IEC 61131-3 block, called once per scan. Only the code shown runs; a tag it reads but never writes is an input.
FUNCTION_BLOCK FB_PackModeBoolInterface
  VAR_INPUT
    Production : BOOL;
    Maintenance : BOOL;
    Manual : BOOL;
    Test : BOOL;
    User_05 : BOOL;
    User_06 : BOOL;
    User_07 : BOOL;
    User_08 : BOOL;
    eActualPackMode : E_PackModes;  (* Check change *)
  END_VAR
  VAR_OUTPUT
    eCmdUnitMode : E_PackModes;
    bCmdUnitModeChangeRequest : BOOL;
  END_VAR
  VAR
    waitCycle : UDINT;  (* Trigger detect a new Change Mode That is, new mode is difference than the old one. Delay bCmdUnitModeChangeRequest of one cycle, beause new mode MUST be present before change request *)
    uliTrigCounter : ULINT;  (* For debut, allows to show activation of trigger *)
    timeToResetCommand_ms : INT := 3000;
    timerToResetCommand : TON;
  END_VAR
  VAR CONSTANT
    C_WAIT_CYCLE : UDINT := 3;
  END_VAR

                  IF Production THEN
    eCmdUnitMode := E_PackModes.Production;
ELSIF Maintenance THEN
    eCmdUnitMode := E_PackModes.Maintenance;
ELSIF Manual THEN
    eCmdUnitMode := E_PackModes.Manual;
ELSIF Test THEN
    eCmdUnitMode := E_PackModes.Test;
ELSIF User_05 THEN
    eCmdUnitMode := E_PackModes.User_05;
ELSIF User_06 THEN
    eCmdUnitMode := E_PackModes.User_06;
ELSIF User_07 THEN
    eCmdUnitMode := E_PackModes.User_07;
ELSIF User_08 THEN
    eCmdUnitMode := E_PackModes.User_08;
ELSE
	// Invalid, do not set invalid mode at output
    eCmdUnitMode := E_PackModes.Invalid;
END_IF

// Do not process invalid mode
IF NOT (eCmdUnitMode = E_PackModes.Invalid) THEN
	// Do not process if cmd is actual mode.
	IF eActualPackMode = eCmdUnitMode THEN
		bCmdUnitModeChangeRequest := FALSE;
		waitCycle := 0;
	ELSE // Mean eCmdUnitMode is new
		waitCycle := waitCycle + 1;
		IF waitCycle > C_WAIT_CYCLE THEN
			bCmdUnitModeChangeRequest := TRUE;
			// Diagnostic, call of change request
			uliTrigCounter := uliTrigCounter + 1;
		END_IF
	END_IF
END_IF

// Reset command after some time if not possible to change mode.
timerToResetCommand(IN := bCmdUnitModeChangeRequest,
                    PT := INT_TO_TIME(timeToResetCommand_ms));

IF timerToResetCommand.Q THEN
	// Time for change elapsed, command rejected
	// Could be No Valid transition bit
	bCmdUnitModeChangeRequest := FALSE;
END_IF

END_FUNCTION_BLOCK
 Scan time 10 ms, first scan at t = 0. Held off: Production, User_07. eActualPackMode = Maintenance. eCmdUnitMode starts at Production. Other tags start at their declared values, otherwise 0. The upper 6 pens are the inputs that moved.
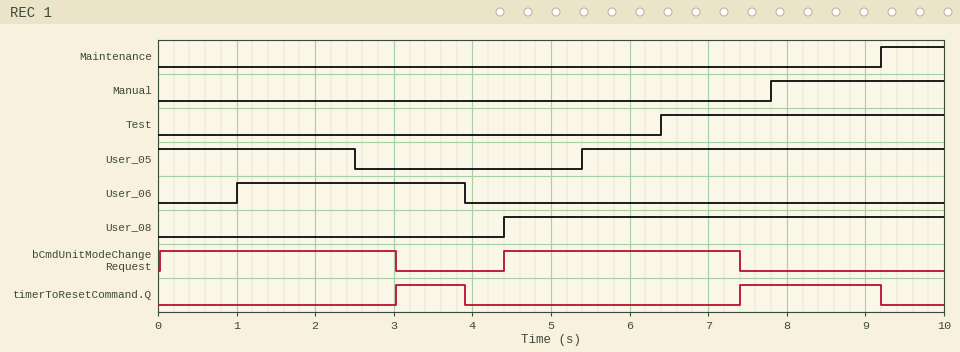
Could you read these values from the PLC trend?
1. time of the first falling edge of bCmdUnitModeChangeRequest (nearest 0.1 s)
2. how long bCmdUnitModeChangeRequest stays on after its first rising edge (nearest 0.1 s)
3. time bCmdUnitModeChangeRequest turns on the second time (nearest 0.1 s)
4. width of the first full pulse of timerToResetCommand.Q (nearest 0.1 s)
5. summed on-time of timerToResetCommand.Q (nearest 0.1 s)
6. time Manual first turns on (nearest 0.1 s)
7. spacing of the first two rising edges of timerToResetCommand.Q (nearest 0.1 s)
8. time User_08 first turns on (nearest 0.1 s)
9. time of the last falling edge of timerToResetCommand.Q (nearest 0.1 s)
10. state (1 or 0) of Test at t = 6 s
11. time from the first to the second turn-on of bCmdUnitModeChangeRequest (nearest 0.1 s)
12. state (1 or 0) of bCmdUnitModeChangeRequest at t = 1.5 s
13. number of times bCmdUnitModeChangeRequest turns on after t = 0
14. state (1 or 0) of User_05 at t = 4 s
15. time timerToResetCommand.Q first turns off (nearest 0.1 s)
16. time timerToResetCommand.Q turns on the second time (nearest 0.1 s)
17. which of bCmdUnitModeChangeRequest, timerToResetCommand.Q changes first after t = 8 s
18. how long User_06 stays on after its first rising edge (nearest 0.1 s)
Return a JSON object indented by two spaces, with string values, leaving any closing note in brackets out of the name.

{
  "time of the first falling edge of bCmdUnitModeChangeRequest": "3.0 s",
  "how long bCmdUnitModeChangeRequest stays on after its first rising edge": "3.0 s",
  "time bCmdUnitModeChangeRequest turns on the second time": "4.4 s",
  "width of the first full pulse of timerToResetCommand.Q": "0.9 s",
  "summed on-time of timerToResetCommand.Q": "2.7 s",
  "time Manual first turns on": "7.8 s",
  "spacing of the first two rising edges of timerToResetCommand.Q": "4.4 s",
  "time User_08 first turns on": "4.4 s",
  "time of the last falling edge of timerToResetCommand.Q": "9.2 s",
  "state (1 or 0) of Test at t = 6 s": "0",
  "time from the first to the second turn-on of bCmdUnitModeChangeRequest": "4.4 s",
  "state (1 or 0) of bCmdUnitModeChangeRequest at t = 1.5 s": "1",
  "number of times bCmdUnitModeChangeRequest turns on after t = 0": "2",
  "state (1 or 0) of User_05 at t = 4 s": "0",
  "time timerToResetCommand.Q first turns off": "3.9 s",
  "time timerToResetCommand.Q turns on the second time": "7.4 s",
  "which of bCmdUnitModeChangeRequest, timerToResetCommand.Q changes first after t = 8 s": "timerToResetCommand.Q",
  "how long User_06 stays on after its first rising edge": "2.9 s"
}
